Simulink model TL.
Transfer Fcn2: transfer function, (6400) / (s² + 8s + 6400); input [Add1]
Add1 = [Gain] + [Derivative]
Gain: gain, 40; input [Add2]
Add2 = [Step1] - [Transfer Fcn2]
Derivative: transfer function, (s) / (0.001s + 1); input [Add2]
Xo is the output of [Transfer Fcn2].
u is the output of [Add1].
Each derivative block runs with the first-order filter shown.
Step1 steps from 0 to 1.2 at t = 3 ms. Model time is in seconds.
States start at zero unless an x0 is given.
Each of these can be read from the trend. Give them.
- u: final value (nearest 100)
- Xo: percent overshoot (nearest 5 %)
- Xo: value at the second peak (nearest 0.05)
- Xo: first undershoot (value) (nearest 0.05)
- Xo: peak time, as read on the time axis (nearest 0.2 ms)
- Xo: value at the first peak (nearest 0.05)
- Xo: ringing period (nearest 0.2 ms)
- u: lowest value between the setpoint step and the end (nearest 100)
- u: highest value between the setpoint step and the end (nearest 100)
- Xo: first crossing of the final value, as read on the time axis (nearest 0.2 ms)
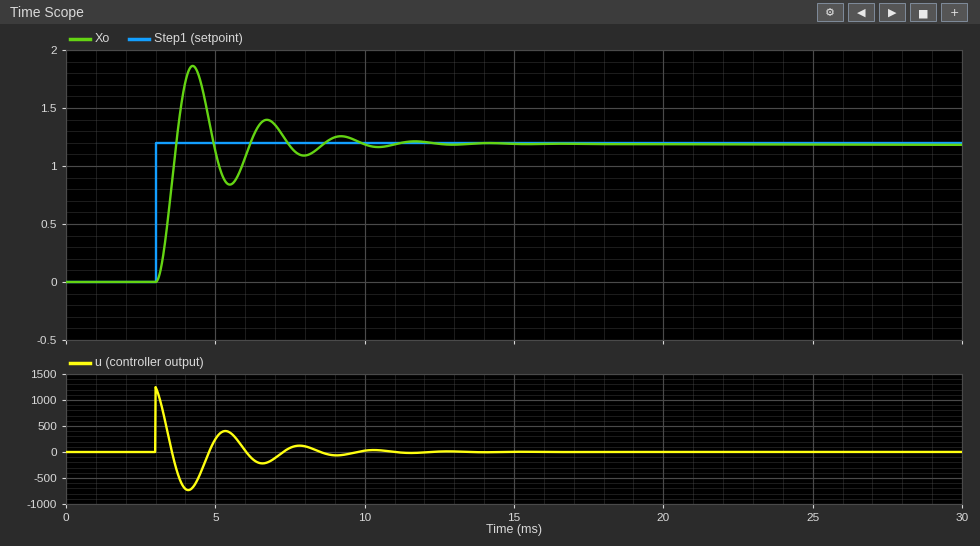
0
60 %
1.40
0.85
4.2 ms
1.85
2.4 ms
-700
1200
3.6 ms
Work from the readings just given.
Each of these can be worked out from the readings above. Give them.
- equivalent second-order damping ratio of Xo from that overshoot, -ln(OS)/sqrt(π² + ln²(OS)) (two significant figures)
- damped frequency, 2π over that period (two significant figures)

0.16
2.6 rad/ms
